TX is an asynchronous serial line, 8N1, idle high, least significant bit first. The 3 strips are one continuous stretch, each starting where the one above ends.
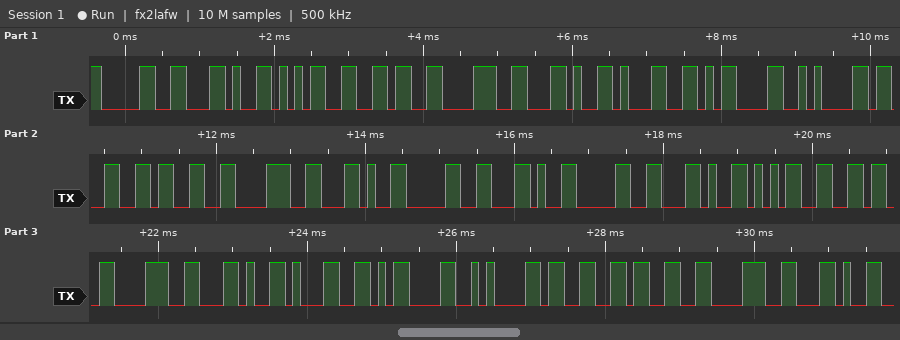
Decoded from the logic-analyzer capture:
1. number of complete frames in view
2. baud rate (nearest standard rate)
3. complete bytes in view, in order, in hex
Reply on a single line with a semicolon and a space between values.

28; 9600 baud; 0x30 0x2C 0x35 0x36 0x38 0x2C 0x31 0x0D 0x0A 0x33 0x33 0x38 0x2C 0x30 0x2C 0x30 0x2C 0x35 0x36 0x38 0x2C 0x31 0x0D 0x0A 0x33 0x33 0x38 0x2C
